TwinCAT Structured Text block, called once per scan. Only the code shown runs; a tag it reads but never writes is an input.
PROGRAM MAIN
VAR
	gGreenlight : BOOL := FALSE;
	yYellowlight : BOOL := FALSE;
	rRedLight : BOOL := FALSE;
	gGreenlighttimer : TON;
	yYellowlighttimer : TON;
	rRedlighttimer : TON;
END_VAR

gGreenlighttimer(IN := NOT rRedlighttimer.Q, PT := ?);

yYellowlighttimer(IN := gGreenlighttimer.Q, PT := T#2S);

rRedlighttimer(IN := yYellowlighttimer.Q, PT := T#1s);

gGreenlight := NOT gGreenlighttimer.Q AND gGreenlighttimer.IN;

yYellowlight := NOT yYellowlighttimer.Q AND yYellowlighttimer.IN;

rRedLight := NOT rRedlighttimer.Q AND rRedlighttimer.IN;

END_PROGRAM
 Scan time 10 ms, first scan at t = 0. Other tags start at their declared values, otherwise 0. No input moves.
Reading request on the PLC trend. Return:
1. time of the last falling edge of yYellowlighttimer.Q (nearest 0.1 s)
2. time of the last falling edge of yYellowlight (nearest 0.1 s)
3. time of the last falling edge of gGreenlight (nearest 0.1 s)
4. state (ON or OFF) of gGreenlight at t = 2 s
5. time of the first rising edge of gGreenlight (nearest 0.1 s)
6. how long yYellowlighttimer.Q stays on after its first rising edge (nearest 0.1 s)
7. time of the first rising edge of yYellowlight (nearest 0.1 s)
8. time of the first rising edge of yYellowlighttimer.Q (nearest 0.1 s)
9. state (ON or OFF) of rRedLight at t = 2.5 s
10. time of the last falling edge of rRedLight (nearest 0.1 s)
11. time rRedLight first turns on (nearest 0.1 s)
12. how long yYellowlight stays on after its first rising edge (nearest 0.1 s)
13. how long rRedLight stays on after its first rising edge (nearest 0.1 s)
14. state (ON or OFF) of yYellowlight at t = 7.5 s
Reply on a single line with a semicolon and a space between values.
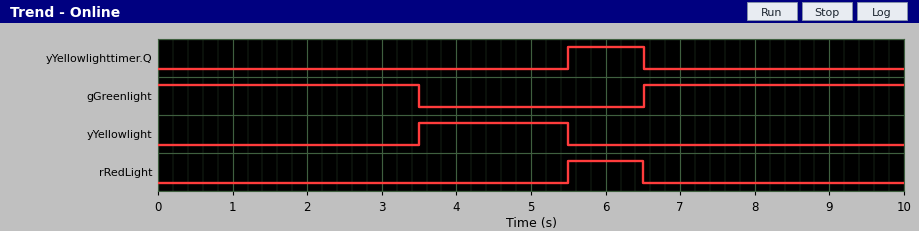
6.5 s; 5.5 s; 3.5 s; ON; 6.5 s; 1.0 s; 3.5 s; 5.5 s; OFF; 6.5 s; 5.5 s; 2.0 s; 1.0 s; OFF
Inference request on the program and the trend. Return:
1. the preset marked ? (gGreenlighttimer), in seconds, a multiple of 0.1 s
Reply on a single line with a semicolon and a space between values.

3.5 s
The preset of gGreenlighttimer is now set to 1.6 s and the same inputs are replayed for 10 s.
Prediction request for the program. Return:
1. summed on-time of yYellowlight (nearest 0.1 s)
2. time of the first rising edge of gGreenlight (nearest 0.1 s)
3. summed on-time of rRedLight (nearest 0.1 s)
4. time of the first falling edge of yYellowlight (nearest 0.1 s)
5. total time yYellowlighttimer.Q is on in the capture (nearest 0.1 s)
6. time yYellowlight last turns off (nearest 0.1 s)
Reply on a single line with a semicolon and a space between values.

4.0 s; 4.6 s; 2.0 s; 3.6 s; 2.0 s; 8.2 s
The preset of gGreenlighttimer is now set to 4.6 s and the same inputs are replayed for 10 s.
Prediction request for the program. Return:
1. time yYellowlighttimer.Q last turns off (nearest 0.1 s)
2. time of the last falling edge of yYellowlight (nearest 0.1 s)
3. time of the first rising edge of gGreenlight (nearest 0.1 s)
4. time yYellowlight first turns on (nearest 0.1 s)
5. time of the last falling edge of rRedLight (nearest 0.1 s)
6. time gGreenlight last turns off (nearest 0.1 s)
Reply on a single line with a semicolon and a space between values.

7.6 s; 6.6 s; 7.6 s; 4.6 s; 7.6 s; 4.6 s
